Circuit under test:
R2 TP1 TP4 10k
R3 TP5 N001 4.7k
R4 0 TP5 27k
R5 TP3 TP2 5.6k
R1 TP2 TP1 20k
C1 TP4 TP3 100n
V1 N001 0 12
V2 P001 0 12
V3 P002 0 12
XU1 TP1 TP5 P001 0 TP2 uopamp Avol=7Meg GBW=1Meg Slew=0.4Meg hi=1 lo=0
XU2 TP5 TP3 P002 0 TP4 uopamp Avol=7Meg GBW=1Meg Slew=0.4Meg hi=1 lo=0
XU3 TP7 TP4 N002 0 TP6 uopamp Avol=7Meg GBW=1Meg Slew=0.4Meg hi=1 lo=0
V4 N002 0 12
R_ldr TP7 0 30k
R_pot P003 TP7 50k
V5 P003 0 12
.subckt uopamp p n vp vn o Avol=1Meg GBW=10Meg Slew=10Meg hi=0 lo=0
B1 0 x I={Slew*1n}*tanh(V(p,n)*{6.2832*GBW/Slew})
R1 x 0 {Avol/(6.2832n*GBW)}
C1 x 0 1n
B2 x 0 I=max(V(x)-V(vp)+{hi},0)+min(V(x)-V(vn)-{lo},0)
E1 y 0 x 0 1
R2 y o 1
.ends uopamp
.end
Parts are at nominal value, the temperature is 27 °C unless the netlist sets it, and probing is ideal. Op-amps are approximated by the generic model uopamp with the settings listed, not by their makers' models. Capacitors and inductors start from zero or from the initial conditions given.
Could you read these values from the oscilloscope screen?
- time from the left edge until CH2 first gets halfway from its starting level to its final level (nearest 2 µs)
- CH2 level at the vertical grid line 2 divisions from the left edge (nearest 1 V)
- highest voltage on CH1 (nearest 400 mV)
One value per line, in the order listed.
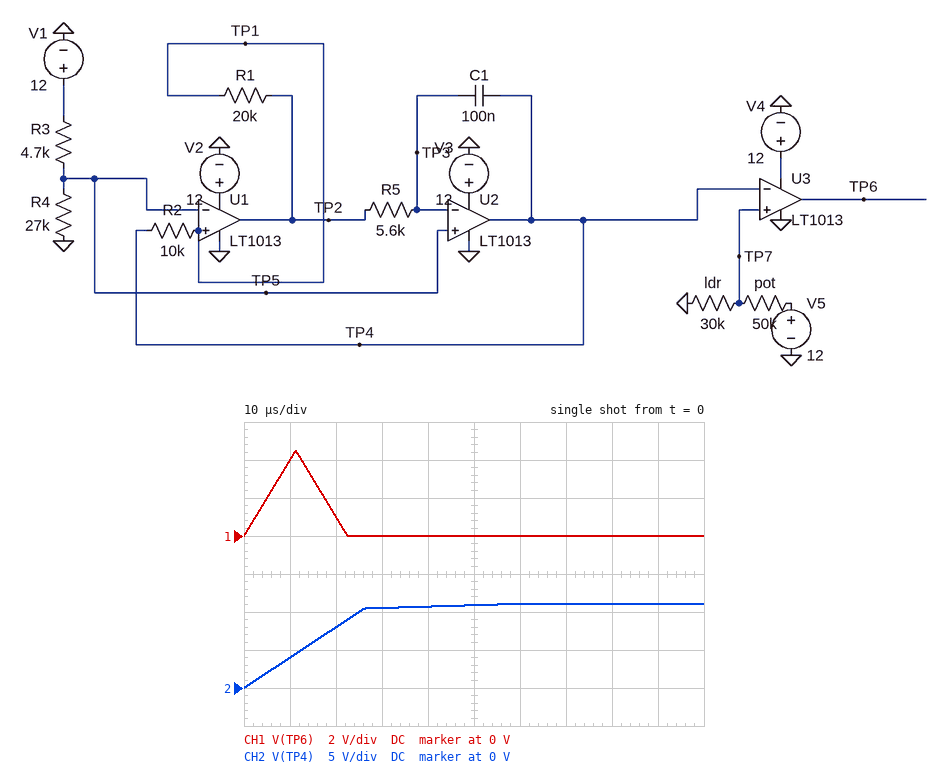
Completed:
14 µs
8 V
4.4 V
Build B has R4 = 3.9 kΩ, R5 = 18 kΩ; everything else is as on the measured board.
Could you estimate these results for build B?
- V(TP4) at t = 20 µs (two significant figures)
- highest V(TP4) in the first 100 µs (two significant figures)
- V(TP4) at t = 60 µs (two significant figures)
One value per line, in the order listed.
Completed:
5.5 V
5.7 V
5.6 V
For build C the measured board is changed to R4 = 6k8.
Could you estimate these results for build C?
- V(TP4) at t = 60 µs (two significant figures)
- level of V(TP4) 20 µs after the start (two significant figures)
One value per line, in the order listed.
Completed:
7.7 V
7.2 V
